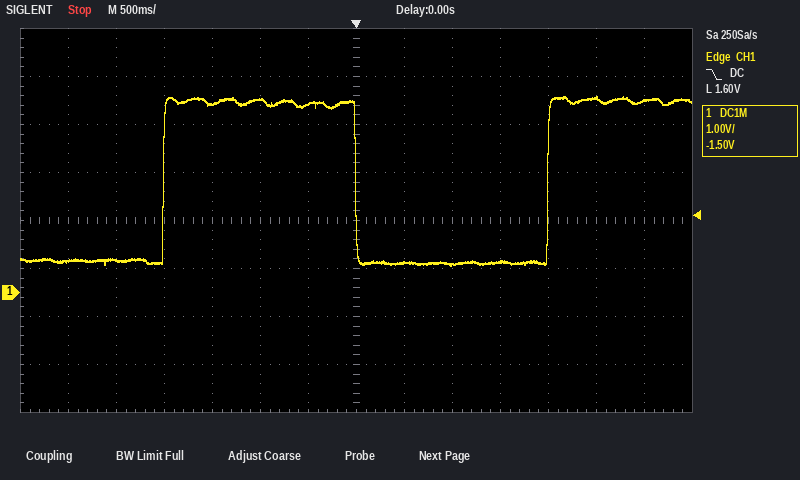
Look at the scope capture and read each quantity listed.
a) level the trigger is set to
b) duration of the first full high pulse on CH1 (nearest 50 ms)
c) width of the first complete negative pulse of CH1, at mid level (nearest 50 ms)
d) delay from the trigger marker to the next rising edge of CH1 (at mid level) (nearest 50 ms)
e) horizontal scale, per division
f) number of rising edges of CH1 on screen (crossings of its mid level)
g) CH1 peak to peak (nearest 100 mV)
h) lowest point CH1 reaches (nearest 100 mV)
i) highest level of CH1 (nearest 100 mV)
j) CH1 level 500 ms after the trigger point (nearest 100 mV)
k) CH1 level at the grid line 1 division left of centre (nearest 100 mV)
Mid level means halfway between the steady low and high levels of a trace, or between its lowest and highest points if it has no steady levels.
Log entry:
1.60 V
2.00 s
2.00 s
2.00 s
500 ms
2
3.5 V
600 mV
4.1 V
600 mV
3.9 V
